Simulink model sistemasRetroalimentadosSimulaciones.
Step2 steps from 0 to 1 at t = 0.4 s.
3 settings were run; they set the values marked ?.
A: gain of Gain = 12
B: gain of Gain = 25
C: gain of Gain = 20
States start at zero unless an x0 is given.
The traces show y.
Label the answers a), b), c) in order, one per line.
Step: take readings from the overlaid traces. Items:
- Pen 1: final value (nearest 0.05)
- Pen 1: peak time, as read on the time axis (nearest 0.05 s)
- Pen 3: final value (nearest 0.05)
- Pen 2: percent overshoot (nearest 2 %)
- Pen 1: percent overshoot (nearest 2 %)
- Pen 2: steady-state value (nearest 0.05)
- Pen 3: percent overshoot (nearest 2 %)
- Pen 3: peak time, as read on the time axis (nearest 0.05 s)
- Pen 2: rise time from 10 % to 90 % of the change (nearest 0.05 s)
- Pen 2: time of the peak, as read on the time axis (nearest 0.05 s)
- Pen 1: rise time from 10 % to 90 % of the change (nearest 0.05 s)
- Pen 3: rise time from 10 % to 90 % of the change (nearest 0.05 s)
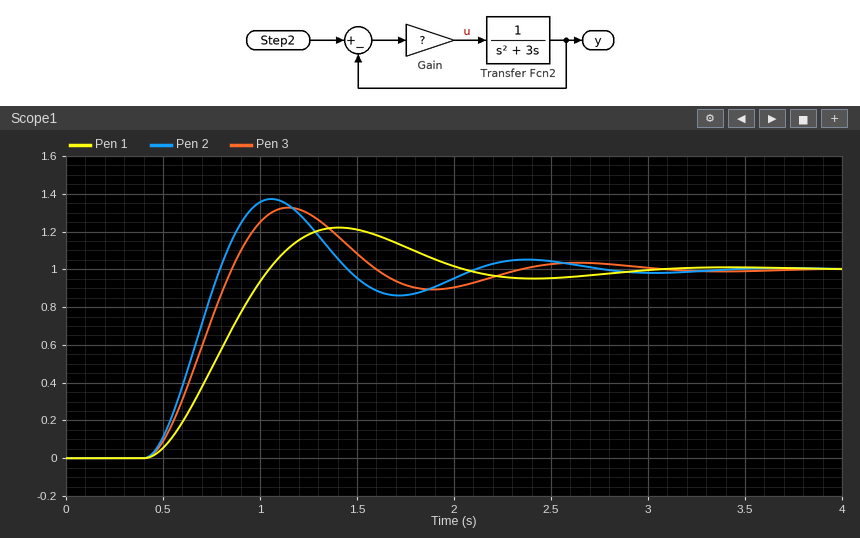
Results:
a) 1.00
b) 1.40 s
c) 1.00
d) 38 %
e) 22 %
f) 1.00
g) 32 %
h) 1.15 s
i) 0.25 s
j) 1.05 s
k) 0.45 s
l) 0.30 s
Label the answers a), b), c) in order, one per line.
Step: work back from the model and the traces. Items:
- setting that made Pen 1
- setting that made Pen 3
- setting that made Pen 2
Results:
a) A
b) C
c) B
